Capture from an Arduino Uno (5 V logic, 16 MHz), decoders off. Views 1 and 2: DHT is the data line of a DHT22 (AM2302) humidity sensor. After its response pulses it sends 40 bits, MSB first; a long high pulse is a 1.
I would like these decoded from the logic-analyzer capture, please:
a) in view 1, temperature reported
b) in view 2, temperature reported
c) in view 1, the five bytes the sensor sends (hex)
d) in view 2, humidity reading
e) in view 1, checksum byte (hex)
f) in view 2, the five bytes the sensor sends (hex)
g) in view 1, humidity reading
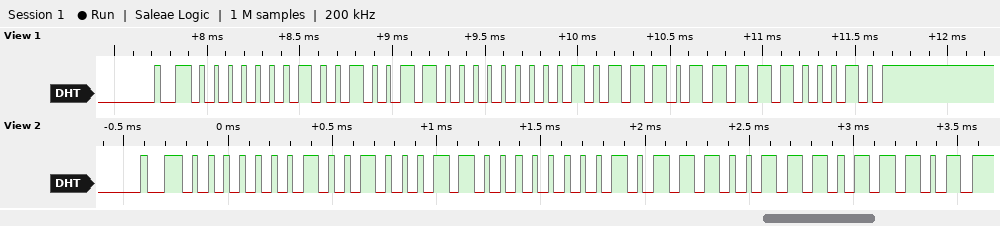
18.7 °C
18.5 °C
01 26 00 BB E2
29.1 %
0xE2
01 23 00 B9 DD
29.4 %
